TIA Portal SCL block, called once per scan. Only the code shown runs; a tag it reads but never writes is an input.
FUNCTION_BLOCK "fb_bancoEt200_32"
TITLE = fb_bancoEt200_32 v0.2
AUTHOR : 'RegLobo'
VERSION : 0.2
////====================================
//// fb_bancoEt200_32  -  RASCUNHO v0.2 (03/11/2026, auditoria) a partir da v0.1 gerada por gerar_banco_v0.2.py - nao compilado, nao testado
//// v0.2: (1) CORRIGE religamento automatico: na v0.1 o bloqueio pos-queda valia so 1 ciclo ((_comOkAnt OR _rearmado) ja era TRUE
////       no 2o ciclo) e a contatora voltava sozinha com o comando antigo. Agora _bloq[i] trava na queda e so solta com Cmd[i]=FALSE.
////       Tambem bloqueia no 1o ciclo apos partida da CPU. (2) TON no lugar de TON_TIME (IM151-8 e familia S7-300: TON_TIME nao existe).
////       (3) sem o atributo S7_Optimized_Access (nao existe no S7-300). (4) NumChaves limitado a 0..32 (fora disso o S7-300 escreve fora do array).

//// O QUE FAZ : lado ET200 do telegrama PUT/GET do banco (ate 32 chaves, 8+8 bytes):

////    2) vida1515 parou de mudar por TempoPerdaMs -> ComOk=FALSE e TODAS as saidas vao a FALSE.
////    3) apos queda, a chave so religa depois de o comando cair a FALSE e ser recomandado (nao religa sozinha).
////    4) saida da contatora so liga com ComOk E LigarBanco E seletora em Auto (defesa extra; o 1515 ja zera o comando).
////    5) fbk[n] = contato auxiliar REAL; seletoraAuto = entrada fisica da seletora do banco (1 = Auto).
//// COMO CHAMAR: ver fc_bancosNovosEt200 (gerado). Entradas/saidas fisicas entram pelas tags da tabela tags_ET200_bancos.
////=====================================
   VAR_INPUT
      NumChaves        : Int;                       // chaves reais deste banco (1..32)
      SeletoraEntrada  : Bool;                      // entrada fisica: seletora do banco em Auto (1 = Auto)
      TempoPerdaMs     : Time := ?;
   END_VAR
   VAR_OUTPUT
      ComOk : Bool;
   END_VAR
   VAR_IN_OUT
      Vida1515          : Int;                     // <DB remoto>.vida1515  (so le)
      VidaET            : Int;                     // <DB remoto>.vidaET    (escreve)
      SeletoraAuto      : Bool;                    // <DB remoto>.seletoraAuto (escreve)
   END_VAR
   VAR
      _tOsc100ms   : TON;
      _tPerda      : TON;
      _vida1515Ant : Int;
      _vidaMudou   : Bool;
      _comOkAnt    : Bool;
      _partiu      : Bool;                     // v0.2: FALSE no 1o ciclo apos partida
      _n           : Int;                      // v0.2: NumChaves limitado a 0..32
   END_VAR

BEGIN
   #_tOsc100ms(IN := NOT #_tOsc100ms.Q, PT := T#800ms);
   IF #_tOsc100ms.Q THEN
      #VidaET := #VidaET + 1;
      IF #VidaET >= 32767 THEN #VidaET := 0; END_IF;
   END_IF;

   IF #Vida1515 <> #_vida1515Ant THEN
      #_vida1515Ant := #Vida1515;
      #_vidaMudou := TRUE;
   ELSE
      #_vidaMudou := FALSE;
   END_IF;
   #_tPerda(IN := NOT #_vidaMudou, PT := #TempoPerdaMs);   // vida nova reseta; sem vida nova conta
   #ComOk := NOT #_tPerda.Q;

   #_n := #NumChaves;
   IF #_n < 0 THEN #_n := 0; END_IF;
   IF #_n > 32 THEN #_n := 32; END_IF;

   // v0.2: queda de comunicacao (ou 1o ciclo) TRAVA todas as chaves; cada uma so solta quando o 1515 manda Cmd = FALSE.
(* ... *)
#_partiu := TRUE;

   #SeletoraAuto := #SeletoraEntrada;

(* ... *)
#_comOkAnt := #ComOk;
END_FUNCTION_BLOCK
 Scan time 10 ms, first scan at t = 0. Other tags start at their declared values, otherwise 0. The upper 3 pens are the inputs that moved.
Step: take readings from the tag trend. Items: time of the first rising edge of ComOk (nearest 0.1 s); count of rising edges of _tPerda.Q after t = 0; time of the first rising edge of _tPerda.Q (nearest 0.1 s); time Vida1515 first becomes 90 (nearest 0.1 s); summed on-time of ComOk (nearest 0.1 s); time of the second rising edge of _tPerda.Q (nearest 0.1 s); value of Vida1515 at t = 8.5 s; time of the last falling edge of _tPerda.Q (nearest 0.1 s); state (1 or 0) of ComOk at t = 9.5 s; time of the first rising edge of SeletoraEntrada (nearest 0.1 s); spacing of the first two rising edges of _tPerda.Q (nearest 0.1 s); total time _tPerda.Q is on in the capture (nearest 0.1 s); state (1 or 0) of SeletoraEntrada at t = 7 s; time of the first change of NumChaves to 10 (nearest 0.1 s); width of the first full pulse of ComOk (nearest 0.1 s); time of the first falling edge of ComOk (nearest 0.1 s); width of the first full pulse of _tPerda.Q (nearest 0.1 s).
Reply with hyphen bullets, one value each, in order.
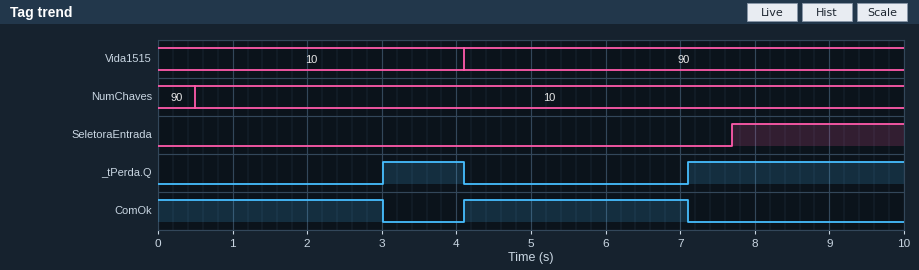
- 4.1 s
- 2
- 3.0 s
- 4.1 s
- 6.0 s
- 7.1 s
- 90
- 4.1 s
- 0
- 7.7 s
- 4.1 s
- 4.0 s
- 0
- 0.5 s
- 3.0 s
- 3.0 s
- 1.1 s
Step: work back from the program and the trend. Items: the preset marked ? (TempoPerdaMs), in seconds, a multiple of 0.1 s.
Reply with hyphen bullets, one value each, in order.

- 3.0 s
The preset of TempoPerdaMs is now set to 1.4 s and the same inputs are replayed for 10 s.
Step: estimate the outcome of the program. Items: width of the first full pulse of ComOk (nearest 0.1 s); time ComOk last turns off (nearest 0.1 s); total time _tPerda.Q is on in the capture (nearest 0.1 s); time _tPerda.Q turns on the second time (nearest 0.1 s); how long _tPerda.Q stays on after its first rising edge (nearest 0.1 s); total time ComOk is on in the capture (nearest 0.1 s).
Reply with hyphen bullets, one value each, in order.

- 1.4 s
- 5.5 s
- 7.2 s
- 5.5 s
- 2.7 s
- 2.8 s
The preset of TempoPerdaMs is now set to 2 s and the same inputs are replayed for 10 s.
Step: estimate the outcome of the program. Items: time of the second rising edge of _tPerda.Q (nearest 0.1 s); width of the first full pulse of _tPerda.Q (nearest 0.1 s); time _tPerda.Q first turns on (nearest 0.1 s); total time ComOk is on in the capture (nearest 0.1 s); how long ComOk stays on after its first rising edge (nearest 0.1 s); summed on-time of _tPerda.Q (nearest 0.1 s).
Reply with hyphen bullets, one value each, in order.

- 6.1 s
- 2.1 s
- 2.0 s
- 4.0 s
- 2.0 s
- 6.0 s
